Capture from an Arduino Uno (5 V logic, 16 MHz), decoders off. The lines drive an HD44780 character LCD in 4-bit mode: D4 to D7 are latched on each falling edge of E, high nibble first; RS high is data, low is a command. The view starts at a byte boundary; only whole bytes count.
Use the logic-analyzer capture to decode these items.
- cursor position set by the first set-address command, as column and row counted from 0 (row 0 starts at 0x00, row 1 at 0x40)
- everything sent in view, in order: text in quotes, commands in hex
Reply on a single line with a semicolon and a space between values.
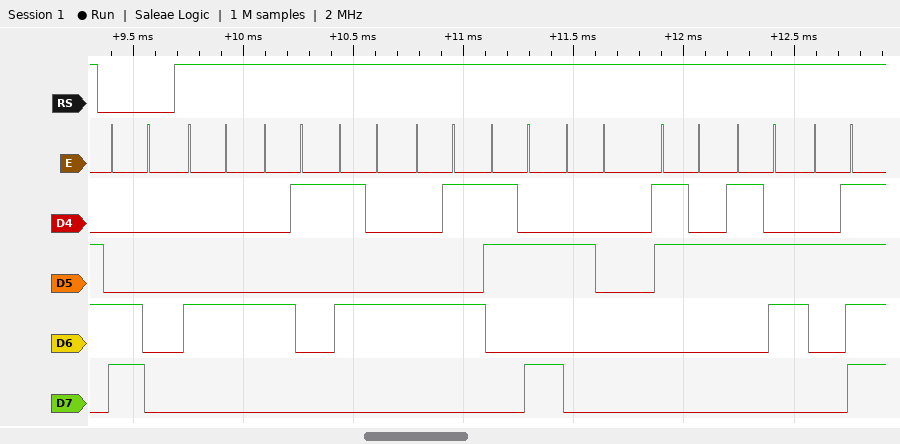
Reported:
column 0, row 1; 0xC0 "DATE: 26/"
